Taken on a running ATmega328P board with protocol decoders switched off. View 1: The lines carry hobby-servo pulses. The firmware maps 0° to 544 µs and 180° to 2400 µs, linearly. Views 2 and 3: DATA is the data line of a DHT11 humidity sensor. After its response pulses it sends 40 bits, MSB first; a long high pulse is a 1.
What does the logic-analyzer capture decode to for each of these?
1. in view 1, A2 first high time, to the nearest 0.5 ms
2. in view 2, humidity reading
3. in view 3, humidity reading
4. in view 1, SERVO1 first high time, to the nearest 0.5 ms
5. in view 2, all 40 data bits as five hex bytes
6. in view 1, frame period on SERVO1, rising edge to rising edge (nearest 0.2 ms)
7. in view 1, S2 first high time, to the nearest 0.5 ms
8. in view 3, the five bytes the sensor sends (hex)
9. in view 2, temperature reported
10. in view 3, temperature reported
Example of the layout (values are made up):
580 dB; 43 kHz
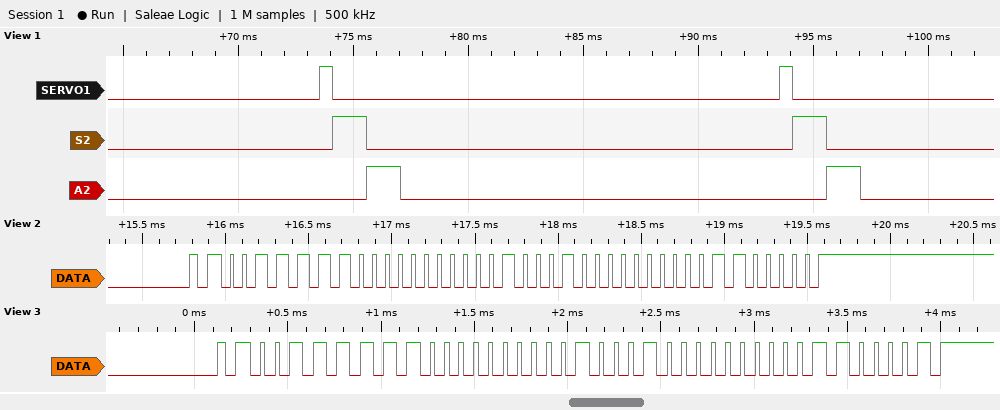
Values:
1.5 ms; 62 %; 63 %; 0.5 ms; 3E 00 22 00 60; 20.0 ms; 1.5 ms; 3F 00 22 00 61; 34.0 °C; 34.0 °C
